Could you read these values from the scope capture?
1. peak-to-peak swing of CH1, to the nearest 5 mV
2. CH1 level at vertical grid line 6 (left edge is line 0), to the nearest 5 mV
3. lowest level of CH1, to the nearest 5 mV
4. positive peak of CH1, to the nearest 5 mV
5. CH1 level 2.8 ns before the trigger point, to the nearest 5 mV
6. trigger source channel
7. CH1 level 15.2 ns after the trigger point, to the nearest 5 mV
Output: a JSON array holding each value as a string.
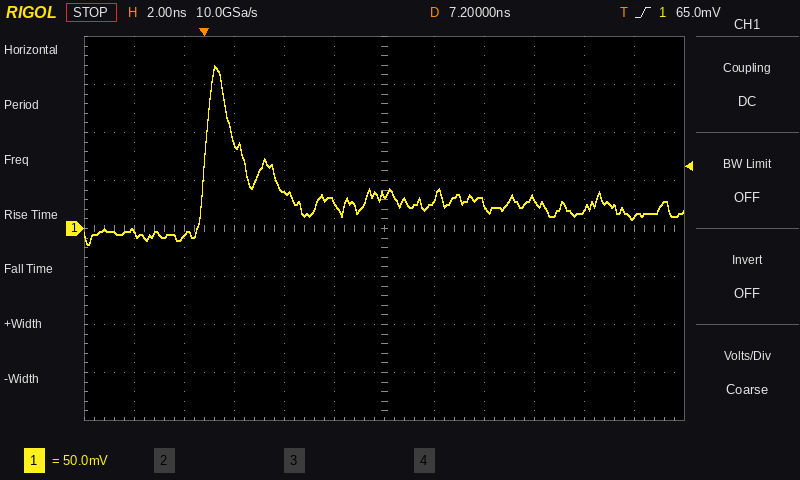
["185 mV", "35 mV", "-15 mV", "170 mV", "-5 mV", "CH1", "20 mV"]
